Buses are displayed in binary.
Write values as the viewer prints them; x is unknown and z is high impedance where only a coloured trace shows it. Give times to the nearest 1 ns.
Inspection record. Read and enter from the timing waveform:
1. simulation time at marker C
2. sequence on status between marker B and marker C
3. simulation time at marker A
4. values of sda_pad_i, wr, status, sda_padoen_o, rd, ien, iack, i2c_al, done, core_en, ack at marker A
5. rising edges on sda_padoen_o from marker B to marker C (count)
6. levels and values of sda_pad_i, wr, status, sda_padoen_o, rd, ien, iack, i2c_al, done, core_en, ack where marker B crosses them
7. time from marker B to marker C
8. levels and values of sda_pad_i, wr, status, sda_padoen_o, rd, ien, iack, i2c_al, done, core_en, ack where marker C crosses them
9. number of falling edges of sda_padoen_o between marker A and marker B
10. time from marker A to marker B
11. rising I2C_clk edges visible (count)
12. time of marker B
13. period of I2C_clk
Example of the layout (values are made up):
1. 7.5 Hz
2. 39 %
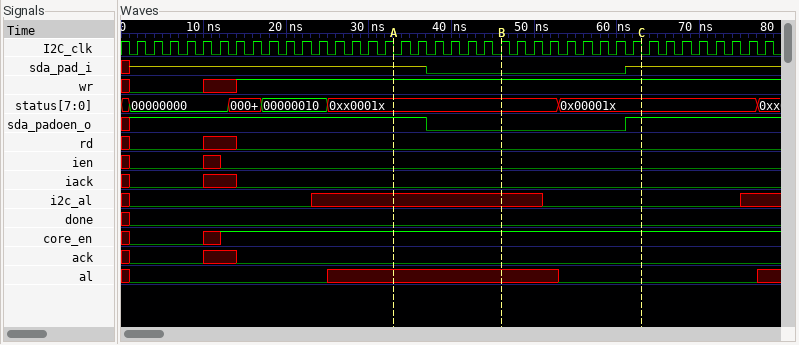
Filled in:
1. 63 ns
2. 0xx0001x, 0x00001x
3. 33 ns
4. sda_pad_i=z, wr=1, status=0xx0001x, sda_padoen_o=1, rd=0, ien=0, iack=0, i2c_al=x, done=0, core_en=1, ack=0
5. 1
6. sda_pad_i=0, wr=1, status=0xx0001x, sda_padoen_o=0, rd=0, ien=0, iack=0, i2c_al=x, done=0, core_en=1, ack=0
7. 17 ns
8. sda_pad_i=z, wr=1, status=0x00001x, sda_padoen_o=1, rd=0, ien=0, iack=0, i2c_al=0, done=0, core_en=1, ack=0
9. 1
10. 13 ns
11. 39
12. 46 ns
13. 2 ns
